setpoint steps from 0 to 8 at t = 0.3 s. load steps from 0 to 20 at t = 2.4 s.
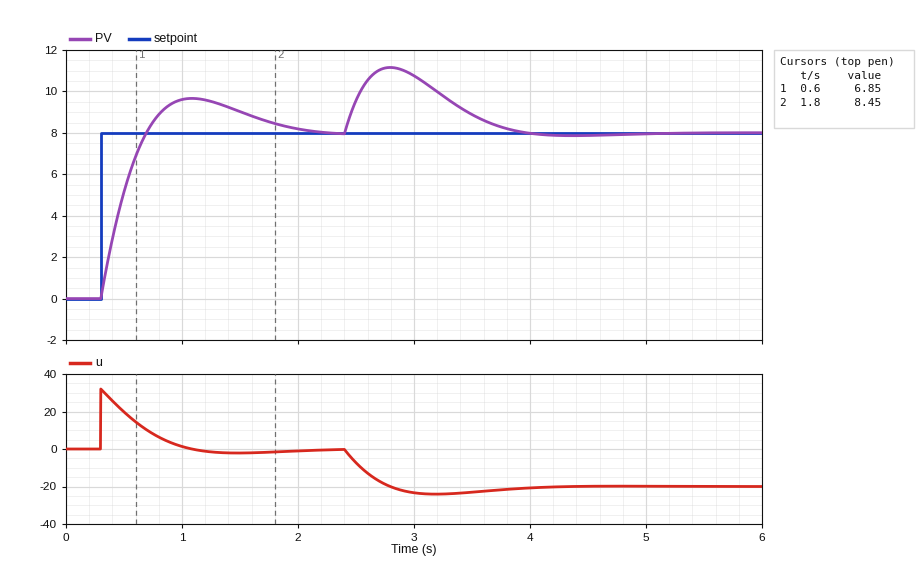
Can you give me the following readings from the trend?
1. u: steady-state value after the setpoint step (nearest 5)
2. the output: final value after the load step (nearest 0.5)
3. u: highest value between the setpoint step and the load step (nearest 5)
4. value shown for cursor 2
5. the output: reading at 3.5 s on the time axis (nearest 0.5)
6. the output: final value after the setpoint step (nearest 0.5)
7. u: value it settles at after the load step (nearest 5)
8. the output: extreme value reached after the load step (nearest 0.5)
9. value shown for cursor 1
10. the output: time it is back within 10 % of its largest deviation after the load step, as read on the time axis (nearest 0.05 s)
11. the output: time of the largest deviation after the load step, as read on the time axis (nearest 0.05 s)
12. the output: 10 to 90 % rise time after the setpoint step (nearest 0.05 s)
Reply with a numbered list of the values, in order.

1. 0
2. 8.0
3. 30
4. 8.45
5. 9.0
6. 8.0
7. -20
8. 11.0
9. 6.85
10. 3.75 s
11. 2.80 s
12. 0.30 s
